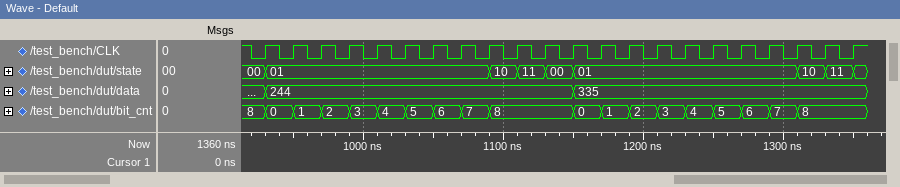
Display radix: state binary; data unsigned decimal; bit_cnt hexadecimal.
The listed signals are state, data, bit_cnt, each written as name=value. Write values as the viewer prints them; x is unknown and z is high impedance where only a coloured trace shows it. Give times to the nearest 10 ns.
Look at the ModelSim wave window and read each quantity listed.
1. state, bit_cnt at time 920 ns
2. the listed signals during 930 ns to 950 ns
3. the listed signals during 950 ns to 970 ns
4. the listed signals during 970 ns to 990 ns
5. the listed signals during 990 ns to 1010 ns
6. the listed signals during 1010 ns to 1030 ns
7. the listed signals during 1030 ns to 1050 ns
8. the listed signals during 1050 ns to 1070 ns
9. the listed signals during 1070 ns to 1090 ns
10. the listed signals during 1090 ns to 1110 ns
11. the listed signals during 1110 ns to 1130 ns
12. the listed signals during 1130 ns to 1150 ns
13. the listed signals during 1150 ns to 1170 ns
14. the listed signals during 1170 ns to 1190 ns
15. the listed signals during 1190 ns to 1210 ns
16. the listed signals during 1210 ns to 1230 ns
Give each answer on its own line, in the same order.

state=00, bit_cnt=8
state=01, data=244, bit_cnt=0
state=01, data=244, bit_cnt=1
state=01, data=244, bit_cnt=2
state=01, data=244, bit_cnt=3
state=01, data=244, bit_cnt=4
state=01, data=244, bit_cnt=5
state=01, data=244, bit_cnt=6
state=01, data=244, bit_cnt=7
state=10, data=244, bit_cnt=8
state=11, data=244, bit_cnt=8
state=00, data=244, bit_cnt=8
state=01, data=335, bit_cnt=0
state=01, data=335, bit_cnt=1
state=01, data=335, bit_cnt=2
state=01, data=335, bit_cnt=3
